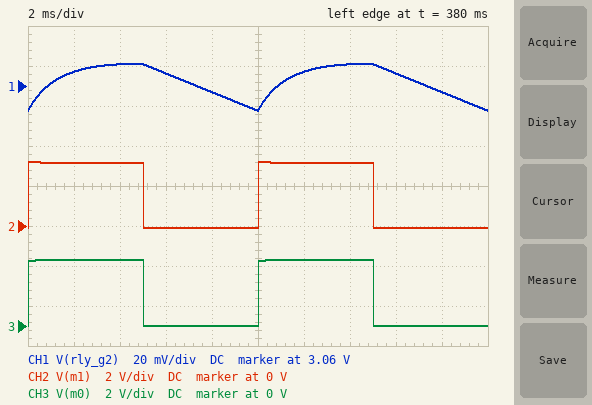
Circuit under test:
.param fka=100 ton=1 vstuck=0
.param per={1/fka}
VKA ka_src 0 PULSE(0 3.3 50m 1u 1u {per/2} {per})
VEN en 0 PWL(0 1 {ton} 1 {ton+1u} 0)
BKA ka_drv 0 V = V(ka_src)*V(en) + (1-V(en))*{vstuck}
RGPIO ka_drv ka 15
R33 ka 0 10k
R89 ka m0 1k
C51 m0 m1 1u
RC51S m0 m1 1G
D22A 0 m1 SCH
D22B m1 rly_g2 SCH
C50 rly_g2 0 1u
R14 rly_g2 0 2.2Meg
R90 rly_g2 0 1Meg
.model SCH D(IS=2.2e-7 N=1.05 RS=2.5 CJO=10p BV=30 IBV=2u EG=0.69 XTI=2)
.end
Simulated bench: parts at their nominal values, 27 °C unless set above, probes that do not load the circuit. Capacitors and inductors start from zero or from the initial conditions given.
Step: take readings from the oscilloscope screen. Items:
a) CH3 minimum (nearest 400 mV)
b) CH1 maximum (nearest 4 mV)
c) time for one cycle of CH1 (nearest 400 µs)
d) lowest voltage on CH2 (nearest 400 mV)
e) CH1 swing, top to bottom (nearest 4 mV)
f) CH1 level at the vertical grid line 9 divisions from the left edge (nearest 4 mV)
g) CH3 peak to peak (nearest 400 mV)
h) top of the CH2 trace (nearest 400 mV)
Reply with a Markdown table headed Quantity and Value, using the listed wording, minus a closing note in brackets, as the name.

| Quantity | Value |
|---|---|
| CH3 minimum | 0 V |
| CH1 maximum | 3.072 V |
| time for one cycle of CH1 | 10.0 ms |
| lowest voltage on CH2 | 0 V |
| CH1 swing, top to bottom | 24 mV |
| CH1 level at the vertical grid line 9 divisions from the left edge | 3.056 V |
| CH3 peak to peak | 3.2 V |
| top of the CH2 trace | 3.2 V |
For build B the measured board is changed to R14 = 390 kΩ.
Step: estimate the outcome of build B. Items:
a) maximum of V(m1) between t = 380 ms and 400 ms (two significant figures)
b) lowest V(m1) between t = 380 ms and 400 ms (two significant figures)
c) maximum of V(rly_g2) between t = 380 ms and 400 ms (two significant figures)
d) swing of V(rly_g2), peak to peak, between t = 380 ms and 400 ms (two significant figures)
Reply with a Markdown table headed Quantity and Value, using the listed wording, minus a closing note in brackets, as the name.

| Quantity | Value |
|---|---|
| maximum of V(m1) between t = 380 ms and 400 ms | 3.1 V |
| lowest V(m1) between t = 380 ms and 400 ms | -150 mV |
| maximum of V(rly_g2) between t = 380 ms and 400 ms | 3.0 V |
| swing of V(rly_g2), peak to peak, between t = 380 ms and 400 ms | 58 mV |
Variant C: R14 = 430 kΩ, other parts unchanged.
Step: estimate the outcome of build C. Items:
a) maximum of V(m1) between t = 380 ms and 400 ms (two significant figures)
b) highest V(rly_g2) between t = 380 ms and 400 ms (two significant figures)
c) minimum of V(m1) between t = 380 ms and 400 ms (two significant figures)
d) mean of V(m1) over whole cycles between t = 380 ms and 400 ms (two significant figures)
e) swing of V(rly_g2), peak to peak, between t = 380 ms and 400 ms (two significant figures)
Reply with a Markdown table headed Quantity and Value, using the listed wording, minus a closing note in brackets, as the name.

| Quantity | Value |
|---|---|
| maximum of V(m1) between t = 380 ms and 400 ms | 3.1 V |
| highest V(rly_g2) between t = 380 ms and 400 ms | 3.0 V |
| minimum of V(m1) between t = 380 ms and 400 ms | -150 mV |
| mean of V(m1) over whole cycles between t = 380 ms and 400 ms | 1.5 V |
| swing of V(rly_g2), peak to peak, between t = 380 ms and 400 ms | 54 mV |
